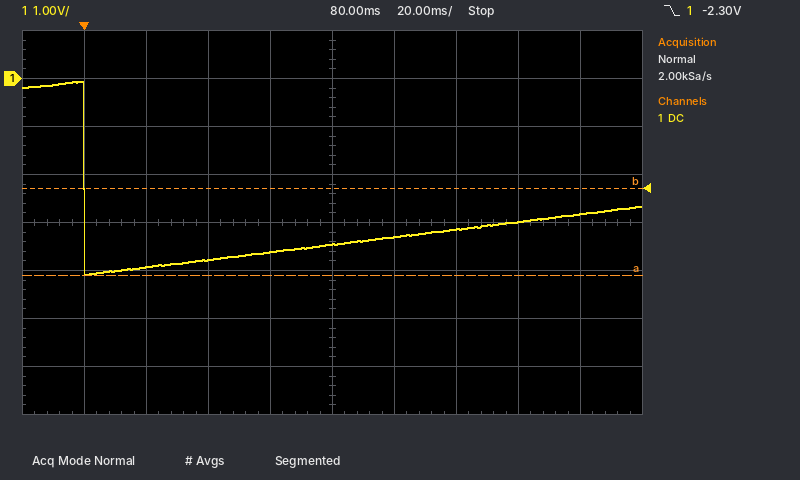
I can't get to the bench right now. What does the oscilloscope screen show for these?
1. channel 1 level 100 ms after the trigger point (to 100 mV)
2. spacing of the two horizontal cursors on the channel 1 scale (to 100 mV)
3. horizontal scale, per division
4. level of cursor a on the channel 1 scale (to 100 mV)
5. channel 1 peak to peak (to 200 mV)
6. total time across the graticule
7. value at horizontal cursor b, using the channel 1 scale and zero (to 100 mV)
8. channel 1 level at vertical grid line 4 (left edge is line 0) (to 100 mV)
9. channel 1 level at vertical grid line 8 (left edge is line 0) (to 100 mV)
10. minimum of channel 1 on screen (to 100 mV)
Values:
-3.3 V
1.8 V
20 ms
-4.1 V
4.0 V
200 ms
-2.3 V
-3.6 V
-3.0 V
-4.1 V
